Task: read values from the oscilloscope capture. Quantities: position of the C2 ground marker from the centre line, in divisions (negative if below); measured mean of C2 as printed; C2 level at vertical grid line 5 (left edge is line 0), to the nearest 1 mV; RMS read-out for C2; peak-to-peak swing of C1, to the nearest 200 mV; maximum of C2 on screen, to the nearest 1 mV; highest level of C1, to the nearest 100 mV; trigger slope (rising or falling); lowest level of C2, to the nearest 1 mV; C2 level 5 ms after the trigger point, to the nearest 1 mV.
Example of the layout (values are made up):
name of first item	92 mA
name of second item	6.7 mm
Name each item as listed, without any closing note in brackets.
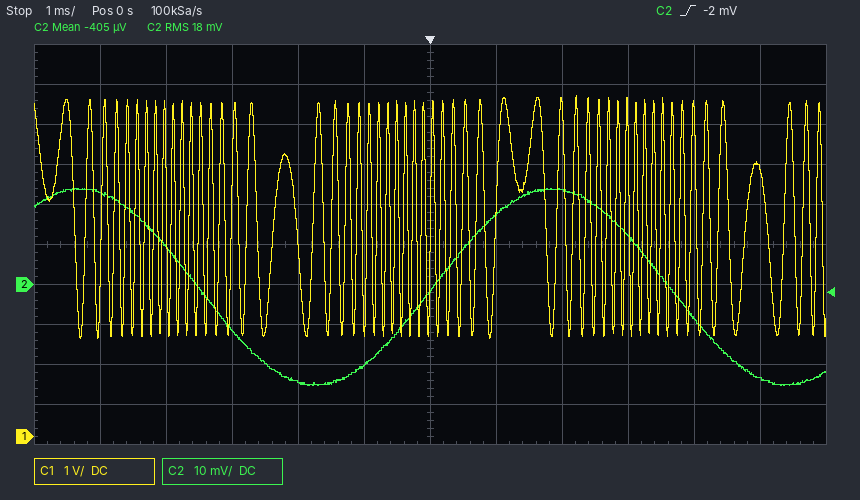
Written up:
position of the C2 ground marker from the centre line, in divisions	-1.0 div
measured mean of C2 as printed	-405 µV
C2 level at vertical grid line 5 (left edge is line 0), to the nearest 1 mV	-20 mV
RMS read-out for C2	18 mV
peak-to-peak swing of C1, to the nearest 200 mV	6.0 V
maximum of C2 on screen, to the nearest 1 mV	24 mV
highest level of C1, to the nearest 100 mV	8.5 V
trigger slope	rising
lowest level of C2, to the nearest 1 mV	-25 mV
C2 level 5 ms after the trigger point, to the nearest 1 mV	-24 mV
